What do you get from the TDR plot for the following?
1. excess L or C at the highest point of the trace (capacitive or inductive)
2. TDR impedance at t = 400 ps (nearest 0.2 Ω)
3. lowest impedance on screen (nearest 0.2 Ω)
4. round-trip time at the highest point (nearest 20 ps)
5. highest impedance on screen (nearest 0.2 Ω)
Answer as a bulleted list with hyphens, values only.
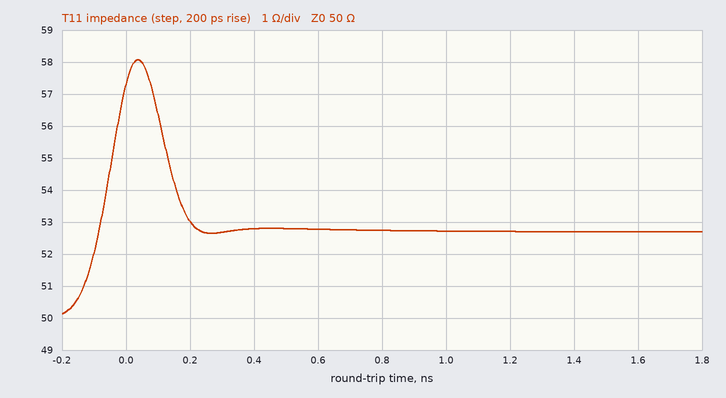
- inductive
- 52.8 Ω
- 50.2 Ω
- 40 ps
- 58.0 Ω
